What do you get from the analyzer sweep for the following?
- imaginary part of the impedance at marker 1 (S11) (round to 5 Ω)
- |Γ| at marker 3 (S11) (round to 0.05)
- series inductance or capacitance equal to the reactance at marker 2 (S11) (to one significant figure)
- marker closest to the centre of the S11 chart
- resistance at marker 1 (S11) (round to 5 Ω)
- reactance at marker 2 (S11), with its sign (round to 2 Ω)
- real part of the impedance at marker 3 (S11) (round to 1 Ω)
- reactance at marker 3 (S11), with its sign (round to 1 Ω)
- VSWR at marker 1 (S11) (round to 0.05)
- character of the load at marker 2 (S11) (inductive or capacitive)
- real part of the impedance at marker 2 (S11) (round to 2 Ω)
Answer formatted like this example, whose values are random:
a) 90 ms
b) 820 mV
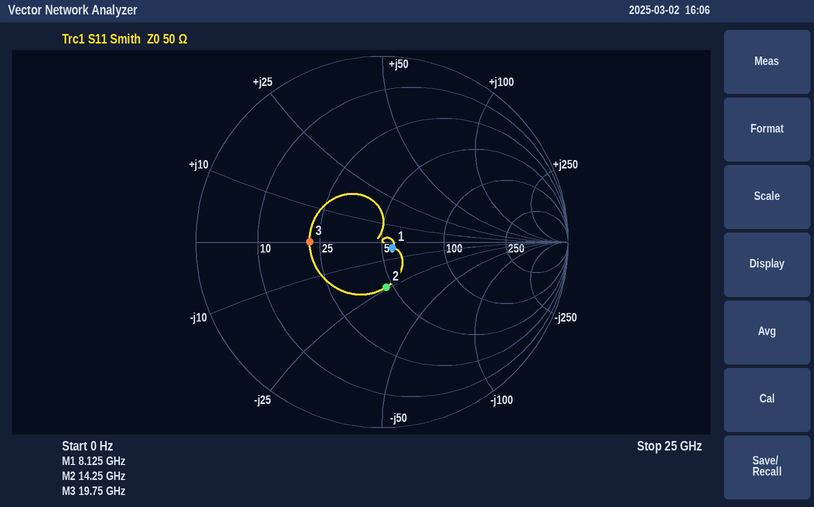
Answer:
a) -5 Ω
b) 0.40
c) 500 fF
d) marker 1
e) 55 Ω
f) -24 Ω
g) 22 Ω
h) 0 Ω
i) 1.15
j) capacitive
k) 46 Ω
